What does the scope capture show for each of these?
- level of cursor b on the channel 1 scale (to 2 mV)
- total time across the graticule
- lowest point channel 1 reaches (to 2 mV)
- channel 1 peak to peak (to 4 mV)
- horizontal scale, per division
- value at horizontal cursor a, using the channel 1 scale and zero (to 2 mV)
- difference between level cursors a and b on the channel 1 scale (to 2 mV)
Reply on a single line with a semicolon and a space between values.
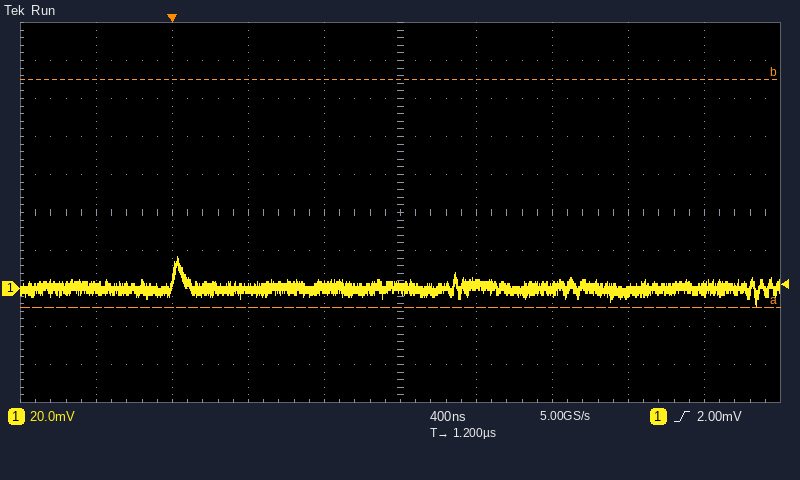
110 mV; 4 µs; -10 mV; 28 mV; 400 ns; -10 mV; 120 mV
